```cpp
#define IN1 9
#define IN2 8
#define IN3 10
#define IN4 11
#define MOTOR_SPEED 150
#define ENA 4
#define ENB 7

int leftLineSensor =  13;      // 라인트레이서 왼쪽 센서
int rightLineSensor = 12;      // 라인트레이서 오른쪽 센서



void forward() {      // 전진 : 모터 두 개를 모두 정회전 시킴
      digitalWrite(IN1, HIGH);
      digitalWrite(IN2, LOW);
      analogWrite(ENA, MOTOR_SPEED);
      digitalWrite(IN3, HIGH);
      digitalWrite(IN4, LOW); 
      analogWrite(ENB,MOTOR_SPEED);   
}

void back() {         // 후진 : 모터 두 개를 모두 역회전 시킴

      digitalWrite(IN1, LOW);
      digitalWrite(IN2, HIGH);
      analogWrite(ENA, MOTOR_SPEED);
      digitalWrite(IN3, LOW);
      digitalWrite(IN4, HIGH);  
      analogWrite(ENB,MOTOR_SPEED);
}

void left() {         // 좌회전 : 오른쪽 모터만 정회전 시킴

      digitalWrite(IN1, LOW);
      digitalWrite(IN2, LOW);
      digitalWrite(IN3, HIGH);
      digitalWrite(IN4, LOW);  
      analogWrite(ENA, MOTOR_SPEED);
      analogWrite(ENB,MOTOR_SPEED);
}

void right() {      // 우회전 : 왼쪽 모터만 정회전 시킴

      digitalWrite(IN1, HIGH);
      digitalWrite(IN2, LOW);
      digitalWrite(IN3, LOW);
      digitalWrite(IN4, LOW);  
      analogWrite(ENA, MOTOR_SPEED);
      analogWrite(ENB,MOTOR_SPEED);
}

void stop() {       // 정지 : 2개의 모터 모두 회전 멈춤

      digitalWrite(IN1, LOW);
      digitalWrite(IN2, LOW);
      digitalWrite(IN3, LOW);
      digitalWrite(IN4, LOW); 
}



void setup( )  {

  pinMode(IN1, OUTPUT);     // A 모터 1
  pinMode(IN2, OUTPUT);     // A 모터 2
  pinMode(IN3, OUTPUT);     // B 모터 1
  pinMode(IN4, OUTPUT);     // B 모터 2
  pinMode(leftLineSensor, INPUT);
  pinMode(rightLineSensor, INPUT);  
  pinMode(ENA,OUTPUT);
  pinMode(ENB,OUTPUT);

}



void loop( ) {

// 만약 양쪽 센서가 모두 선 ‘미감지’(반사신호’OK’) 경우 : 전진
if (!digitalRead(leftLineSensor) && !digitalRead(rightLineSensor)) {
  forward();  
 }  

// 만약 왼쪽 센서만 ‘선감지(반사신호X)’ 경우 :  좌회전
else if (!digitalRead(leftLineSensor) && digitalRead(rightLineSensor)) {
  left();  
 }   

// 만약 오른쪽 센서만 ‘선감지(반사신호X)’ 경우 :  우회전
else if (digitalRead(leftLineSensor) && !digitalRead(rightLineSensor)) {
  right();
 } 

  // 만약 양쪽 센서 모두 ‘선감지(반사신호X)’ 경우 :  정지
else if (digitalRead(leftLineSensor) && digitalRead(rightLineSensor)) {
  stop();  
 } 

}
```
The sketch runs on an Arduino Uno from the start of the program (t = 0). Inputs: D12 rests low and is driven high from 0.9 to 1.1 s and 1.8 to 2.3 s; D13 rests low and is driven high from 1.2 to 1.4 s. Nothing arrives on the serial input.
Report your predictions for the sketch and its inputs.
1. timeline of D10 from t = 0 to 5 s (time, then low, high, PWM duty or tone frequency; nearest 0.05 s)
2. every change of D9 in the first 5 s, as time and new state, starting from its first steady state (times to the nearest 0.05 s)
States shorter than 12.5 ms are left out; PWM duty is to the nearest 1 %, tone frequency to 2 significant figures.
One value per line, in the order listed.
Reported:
0 s high; 1.2 s low; 1.4 s high
0 s high; 0.9 s low; 1.1 s high; 1.8 s low; 2.3 s high
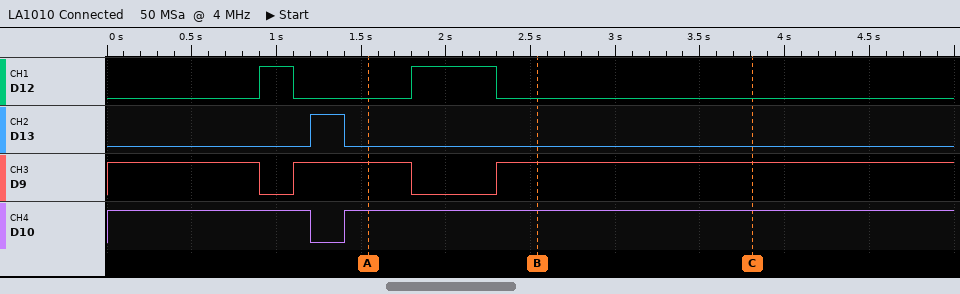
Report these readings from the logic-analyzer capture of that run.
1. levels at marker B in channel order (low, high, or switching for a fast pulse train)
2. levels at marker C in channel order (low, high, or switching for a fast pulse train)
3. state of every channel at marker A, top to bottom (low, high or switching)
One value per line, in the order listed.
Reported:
D12 low, D13 low, D9 high, D10 high
D12 low, D13 low, D9 high, D10 high
D12 low, D13 low, D9 high, D10 high
